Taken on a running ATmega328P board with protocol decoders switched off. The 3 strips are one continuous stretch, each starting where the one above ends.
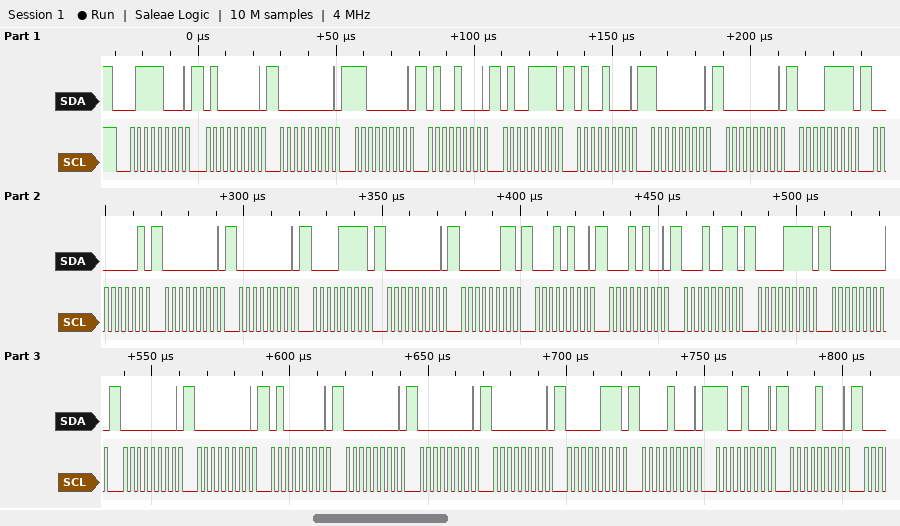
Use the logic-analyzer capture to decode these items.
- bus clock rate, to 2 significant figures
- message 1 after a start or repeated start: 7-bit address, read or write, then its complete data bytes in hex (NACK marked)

400 kHz
0x3C write: 40 00 C0 48 4F 48 80 00 0F 01 00 00 0F 00 03 14 14 13 0F 00 00 00 40 00 00 00 07 08 C8 08
